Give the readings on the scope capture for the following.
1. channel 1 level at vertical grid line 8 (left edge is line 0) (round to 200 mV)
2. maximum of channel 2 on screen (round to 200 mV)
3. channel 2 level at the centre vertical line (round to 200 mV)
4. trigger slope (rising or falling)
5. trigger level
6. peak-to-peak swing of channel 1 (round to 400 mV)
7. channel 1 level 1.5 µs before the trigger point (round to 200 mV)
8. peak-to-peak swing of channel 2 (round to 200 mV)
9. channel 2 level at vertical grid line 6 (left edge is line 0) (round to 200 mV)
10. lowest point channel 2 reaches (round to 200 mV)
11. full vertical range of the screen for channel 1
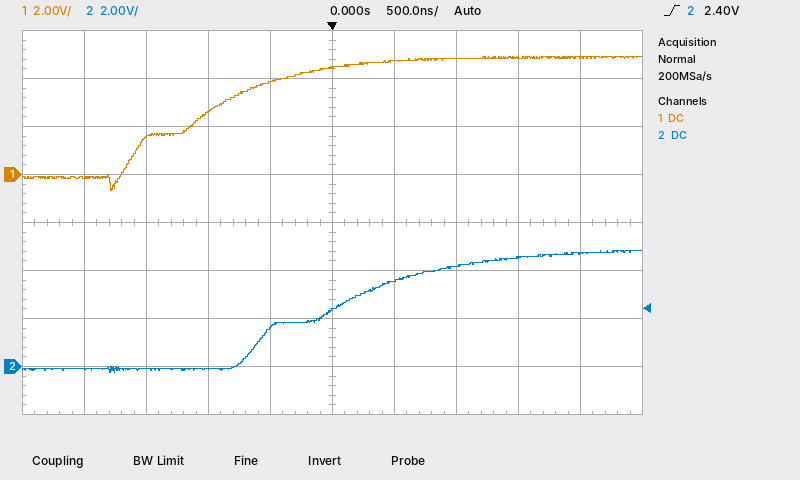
4.8 V
4.8 V
2.4 V
rising
2.40 V
5.6 V
1.6 V
5.0 V
3.6 V
-200 mV
16 V
